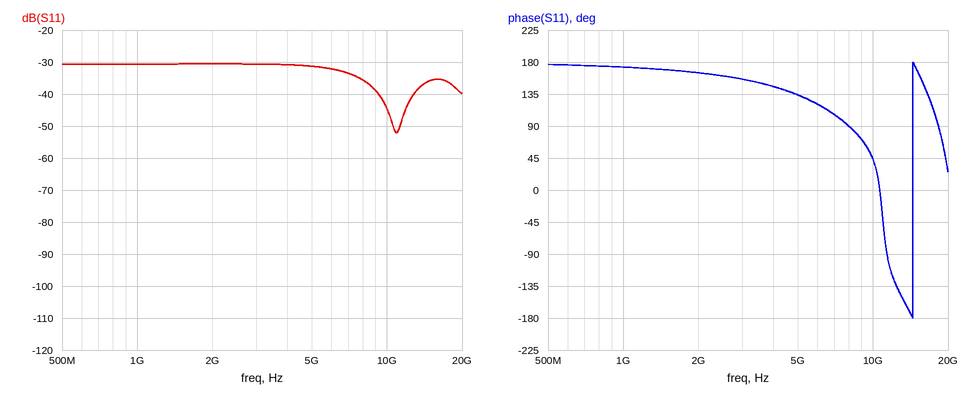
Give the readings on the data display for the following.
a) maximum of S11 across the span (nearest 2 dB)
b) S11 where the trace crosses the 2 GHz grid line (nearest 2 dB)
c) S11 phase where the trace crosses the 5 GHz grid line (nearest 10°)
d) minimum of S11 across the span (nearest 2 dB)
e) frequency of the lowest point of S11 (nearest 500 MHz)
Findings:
-30 dB
-30 dB
130°
-52 dB
11.0 GHz
